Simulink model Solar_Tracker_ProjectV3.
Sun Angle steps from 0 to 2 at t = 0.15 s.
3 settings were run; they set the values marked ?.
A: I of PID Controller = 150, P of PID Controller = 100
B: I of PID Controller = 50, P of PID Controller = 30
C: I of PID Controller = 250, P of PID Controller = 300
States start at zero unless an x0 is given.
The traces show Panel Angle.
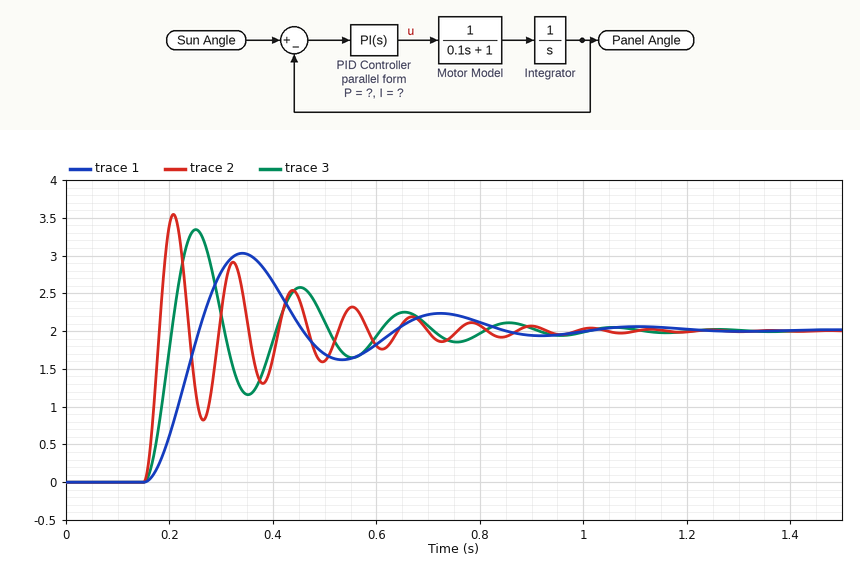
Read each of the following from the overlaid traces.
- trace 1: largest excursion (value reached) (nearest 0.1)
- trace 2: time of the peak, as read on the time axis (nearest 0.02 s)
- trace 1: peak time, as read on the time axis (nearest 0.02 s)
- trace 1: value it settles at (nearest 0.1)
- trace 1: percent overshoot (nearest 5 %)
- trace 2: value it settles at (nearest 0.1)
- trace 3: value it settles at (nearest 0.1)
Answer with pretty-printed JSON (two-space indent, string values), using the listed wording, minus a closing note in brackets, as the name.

{
  "trace 1: largest excursion (value reached)": "3.0",
  "trace 2: time of the peak, as read on the time axis": "0.20 s",
  "trace 1: peak time, as read on the time axis": "0.34 s",
  "trace 1: value it settles at": "2.0",
  "trace 1: percent overshoot": "50 %",
  "trace 2: value it settles at": "2.0",
  "trace 3: value it settles at": "2.0"
}
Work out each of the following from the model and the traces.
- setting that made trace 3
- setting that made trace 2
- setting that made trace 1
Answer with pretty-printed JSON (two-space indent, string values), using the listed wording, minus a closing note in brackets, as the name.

{
  "setting that made trace 3": "A",
  "setting that made trace 2": "C",
  "setting that made trace 1": "B"
}
